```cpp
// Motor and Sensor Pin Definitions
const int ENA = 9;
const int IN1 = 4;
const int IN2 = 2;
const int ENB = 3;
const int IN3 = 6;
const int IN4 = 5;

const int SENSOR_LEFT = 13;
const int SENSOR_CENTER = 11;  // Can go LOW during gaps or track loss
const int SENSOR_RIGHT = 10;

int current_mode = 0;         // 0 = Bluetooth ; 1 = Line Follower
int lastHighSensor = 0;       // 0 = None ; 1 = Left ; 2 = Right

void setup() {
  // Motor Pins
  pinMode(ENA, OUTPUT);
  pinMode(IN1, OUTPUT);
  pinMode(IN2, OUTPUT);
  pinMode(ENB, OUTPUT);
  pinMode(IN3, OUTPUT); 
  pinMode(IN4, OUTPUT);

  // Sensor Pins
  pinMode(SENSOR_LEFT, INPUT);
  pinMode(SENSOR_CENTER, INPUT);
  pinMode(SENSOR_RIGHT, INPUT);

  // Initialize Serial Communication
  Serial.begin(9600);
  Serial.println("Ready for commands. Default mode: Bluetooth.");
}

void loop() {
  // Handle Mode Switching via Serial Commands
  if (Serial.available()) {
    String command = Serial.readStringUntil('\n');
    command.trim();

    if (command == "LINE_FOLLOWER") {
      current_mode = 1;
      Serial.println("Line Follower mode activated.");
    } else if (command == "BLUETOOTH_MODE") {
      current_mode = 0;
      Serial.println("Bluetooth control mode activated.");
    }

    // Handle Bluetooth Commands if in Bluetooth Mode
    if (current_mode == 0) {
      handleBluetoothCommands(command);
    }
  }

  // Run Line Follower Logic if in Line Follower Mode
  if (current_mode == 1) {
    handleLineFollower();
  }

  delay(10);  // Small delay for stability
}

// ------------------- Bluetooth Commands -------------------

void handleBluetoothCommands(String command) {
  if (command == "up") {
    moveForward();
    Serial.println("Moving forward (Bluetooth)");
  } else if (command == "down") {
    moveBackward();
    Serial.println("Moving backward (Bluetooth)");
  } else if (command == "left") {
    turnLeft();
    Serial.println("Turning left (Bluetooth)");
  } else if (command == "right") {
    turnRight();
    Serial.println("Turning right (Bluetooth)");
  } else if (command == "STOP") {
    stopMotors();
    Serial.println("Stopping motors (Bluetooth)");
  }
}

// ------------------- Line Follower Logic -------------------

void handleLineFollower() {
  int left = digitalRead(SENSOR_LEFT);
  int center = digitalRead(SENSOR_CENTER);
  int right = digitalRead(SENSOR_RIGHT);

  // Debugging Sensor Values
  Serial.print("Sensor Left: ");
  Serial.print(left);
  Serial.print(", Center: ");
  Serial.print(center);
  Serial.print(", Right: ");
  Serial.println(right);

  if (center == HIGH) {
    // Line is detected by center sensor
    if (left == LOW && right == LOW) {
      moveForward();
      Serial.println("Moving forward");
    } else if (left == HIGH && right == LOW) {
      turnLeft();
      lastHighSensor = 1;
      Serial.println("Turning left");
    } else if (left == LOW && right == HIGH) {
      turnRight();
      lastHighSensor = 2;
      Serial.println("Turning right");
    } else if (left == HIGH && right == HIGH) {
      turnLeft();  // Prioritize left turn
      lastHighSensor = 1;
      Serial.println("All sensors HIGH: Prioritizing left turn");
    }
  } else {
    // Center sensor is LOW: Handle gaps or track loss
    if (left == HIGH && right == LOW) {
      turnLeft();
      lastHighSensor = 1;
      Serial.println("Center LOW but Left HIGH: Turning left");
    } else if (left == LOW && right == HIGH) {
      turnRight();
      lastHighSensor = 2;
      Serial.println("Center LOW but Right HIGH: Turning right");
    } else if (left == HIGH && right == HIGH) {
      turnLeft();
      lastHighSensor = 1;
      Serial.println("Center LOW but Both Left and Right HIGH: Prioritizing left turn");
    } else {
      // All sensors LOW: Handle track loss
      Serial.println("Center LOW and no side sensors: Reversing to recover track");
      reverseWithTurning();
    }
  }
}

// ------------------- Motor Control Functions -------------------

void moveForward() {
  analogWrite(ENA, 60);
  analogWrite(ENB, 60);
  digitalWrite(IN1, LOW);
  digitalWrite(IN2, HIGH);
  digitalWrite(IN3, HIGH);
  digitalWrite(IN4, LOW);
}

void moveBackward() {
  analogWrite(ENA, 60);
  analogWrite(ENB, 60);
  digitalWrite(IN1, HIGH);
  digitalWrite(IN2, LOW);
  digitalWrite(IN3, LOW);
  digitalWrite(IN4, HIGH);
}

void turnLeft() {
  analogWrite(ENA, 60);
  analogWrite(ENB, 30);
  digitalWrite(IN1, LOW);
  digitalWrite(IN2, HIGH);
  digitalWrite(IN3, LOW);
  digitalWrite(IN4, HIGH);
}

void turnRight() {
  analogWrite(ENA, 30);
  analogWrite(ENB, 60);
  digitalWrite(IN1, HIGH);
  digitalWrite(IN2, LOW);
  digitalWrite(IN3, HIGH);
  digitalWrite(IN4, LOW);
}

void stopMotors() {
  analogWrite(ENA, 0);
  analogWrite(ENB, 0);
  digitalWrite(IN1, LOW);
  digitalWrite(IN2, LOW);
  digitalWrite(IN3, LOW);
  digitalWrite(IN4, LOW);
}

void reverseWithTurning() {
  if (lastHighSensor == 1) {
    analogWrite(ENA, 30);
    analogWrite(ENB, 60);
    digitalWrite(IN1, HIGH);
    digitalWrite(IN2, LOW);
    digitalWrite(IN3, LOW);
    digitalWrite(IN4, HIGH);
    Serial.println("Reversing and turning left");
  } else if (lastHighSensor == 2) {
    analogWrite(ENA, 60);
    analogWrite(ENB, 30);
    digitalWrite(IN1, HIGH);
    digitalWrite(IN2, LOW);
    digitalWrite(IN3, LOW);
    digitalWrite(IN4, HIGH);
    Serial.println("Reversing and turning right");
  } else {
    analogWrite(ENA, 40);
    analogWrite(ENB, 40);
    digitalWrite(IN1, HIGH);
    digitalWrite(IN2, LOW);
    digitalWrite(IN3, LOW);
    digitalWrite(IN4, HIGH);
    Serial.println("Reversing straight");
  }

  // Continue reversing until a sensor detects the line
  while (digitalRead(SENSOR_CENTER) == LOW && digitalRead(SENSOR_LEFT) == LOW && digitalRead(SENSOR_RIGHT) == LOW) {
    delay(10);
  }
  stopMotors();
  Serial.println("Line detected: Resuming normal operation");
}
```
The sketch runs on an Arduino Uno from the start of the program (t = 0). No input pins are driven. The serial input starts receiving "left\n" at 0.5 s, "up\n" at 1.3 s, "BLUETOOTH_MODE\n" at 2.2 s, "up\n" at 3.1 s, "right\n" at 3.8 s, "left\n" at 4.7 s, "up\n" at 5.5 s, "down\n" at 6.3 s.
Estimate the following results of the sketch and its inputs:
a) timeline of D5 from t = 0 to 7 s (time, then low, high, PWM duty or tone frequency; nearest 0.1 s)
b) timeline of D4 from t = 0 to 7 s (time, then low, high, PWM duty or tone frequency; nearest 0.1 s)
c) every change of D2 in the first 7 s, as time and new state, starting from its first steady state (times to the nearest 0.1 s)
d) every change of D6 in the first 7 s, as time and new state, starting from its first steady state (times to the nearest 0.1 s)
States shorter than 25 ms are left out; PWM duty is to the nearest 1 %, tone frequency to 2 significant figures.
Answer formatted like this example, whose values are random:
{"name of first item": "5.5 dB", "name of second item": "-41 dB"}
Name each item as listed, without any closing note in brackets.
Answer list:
{"timeline of D5 from t = 0 to 7 s": "0 s low; 0.5 s high; 1.3 s low; 4.7 s high; 5.5 s low; 6.3 s high", "timeline of D4 from t = 0 to 7 s": "0 s low; 3.8 s high; 4.7 s low; 6.3 s high", "every change of D2 in the first 7 s, as time and new state, starting from its first steady state": "0 s low; 0.5 s high; 3.8 s low; 4.7 s high; 6.3 s low", "every change of D6 in the first 7 s, as time and new state, starting from its first steady state": "0 s low; 1.3 s high; 4.7 s low; 5.5 s high; 6.3 s low"}
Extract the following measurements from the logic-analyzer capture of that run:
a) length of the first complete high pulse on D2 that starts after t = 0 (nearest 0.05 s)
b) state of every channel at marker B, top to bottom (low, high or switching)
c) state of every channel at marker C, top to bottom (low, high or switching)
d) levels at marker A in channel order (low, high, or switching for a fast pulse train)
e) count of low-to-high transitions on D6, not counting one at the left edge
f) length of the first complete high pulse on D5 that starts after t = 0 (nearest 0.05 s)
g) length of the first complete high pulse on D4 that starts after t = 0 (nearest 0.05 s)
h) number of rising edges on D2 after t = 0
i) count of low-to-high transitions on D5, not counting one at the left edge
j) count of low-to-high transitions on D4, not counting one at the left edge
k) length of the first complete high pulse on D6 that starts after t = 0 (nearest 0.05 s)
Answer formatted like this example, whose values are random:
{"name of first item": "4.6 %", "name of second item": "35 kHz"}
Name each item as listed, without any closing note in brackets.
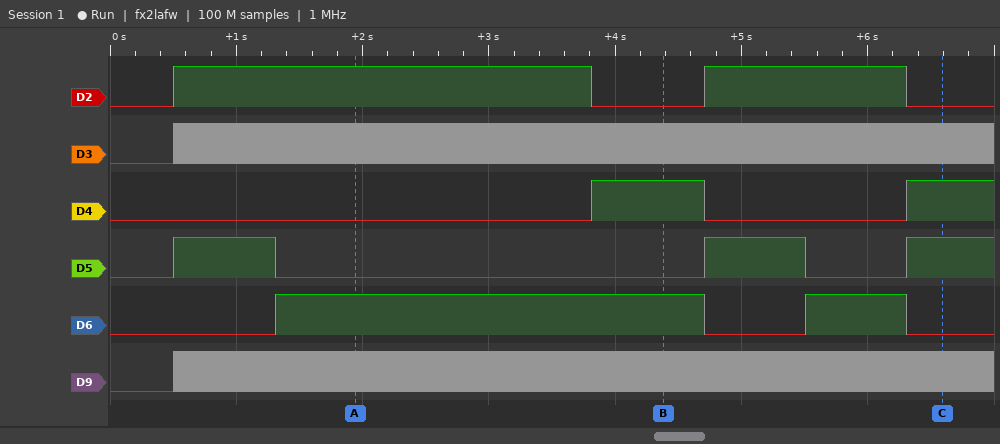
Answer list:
{"length of the first complete high pulse on D2 that starts after t = 0": "3.30 s", "state of every channel at marker B, top to bottom": "D2 low, D3 switching, D4 high, D5 low, D6 high, D9 switching", "state of every channel at marker C, top to bottom": "D2 low, D3 switching, D4 high, D5 high, D6 low, D9 switching", "levels at marker A in channel order": "D2 high, D3 switching, D4 low, D5 low, D6 high, D9 switching", "count of low-to-high transitions on D6, not counting one at the left edge": "2", "length of the first complete high pulse on D5 that starts after t = 0": "0.80 s", "length of the first complete high pulse on D4 that starts after t = 0": "0.90 s", "number of rising edges on D2 after t = 0": "2", "count of low-to-high transitions on D5, not counting one at the left edge": "3", "count of low-to-high transitions on D4, not counting one at the left edge": "2", "length of the first complete high pulse on D6 that starts after t = 0": "3.40 s"}
